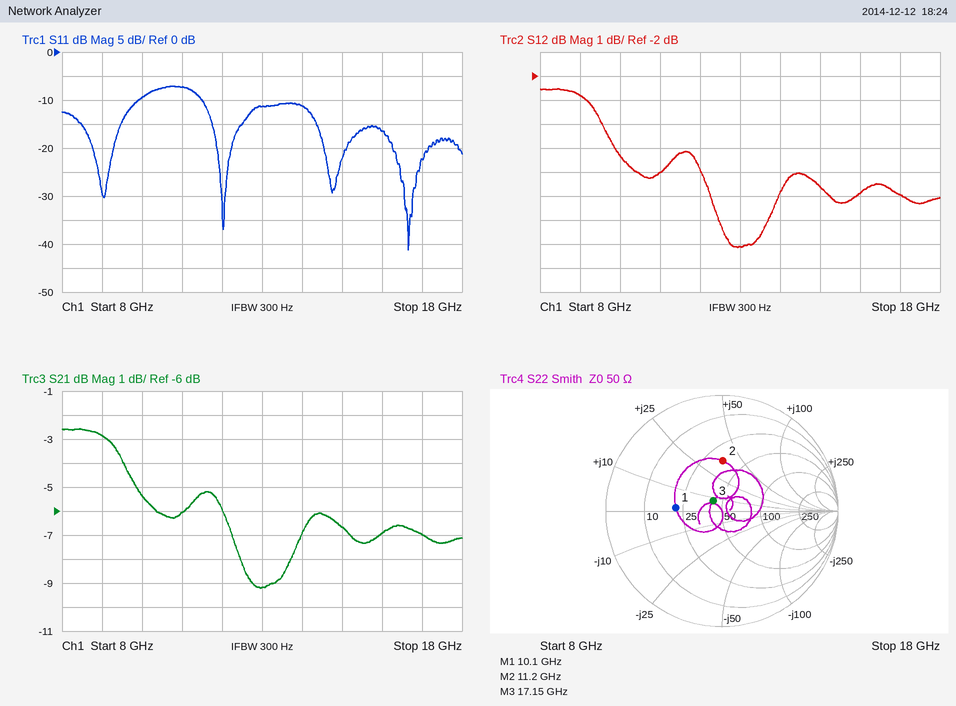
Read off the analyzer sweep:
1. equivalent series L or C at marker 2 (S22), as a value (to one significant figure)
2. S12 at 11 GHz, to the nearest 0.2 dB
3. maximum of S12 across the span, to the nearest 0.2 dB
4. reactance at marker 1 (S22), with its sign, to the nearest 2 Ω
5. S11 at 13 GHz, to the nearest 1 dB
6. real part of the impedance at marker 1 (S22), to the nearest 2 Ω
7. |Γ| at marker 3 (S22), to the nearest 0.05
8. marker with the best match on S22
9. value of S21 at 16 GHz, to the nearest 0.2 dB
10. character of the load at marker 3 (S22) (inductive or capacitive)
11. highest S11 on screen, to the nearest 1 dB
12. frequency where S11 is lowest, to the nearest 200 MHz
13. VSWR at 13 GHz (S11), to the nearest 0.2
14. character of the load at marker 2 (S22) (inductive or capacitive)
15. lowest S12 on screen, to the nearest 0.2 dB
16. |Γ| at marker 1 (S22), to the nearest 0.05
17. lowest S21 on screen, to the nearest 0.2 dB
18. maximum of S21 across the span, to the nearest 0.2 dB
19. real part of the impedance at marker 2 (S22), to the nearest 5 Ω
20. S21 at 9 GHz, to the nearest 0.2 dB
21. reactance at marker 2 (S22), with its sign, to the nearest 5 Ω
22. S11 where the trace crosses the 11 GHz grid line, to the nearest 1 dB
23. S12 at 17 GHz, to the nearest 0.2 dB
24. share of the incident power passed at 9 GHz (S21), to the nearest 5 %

500 pH
-6.0 dB
-2.6 dB
+2 Ω
-11 dB
22 Ω
0.10
marker 3
-7.0 dB
inductive
-7 dB
16.6 GHz
1.8
inductive
-9.2 dB
0.40
-9.2 dB
-2.6 dB
35 Ω
-2.8 dB
+35 Ω
-7 dB
-7.0 dB
50 %
